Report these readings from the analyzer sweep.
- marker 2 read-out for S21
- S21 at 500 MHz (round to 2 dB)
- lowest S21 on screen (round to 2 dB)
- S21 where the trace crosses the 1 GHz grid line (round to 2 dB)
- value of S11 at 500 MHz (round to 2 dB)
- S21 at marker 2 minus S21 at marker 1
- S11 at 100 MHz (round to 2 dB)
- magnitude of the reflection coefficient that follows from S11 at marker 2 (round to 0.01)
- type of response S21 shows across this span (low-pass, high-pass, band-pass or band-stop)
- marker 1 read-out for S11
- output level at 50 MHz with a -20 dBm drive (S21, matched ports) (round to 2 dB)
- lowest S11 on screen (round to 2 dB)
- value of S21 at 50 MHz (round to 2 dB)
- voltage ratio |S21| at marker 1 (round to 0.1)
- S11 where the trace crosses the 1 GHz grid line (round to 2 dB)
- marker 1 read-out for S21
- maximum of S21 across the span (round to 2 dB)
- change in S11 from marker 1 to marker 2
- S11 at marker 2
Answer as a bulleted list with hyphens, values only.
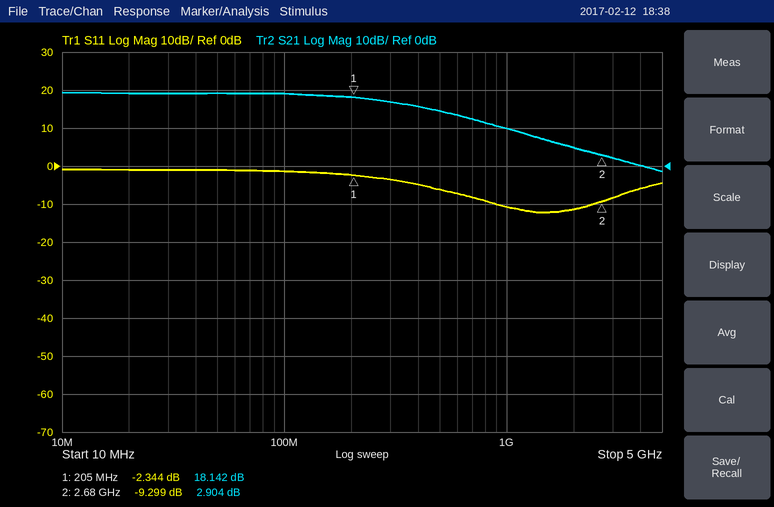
- 2.904 dB
- 14 dB
- -2 dB
- 10 dB
- -6 dB
- -15.238 dB
- -2 dB
- 0.34
- low-pass
- -2.344 dB
- 0 dBm
- -12 dB
- 20 dB
- 8.1
- -10 dB
- 18.142 dB
- 20 dB
- -6.955 dB
- -9.299 dB
